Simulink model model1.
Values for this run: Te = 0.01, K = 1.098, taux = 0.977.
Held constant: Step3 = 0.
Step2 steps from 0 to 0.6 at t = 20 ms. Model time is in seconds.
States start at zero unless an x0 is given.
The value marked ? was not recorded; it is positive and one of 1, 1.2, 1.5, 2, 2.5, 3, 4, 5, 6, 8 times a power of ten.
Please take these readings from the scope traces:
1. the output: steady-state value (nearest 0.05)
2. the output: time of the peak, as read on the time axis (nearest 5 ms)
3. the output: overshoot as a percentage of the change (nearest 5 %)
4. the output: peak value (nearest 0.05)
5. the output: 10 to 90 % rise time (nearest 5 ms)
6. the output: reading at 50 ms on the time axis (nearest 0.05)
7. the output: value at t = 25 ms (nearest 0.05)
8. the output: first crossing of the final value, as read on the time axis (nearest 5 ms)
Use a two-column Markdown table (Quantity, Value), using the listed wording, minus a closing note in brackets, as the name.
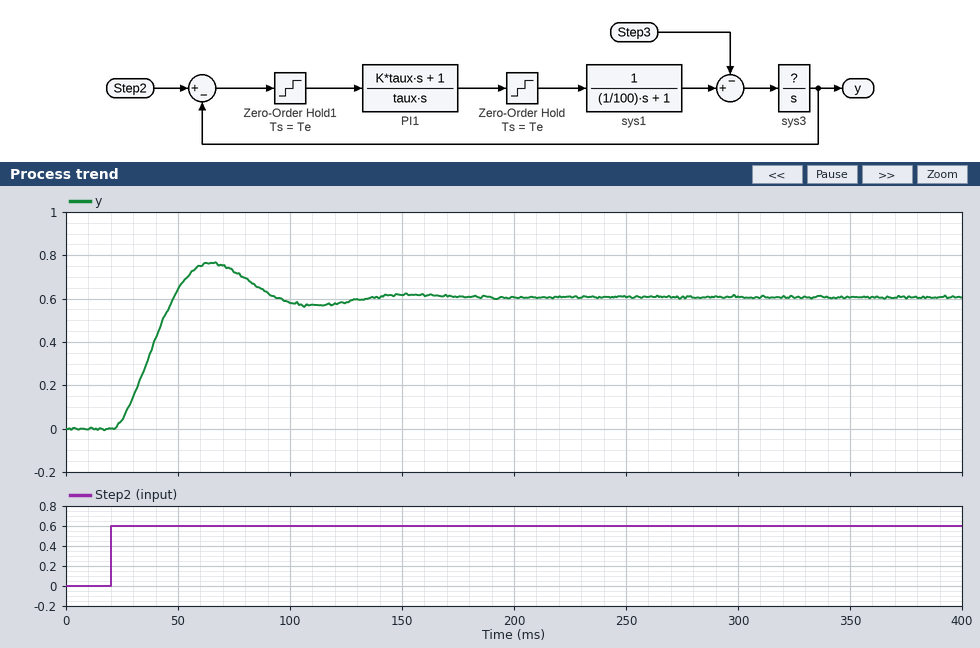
| Quantity | Value |
|---|---|
| the output: steady-state value | 0.60 |
| the output: time of the peak, as read on the time axis | 65 ms |
| the output: overshoot as a percentage of the change | 25 % |
| the output: peak value | 0.75 |
| the output: 10 to 90 % rise time | 20 ms |
| the output: reading at 50 ms on the time axis | 0.65 |
| the output: value at t = 25 ms | 0.05 |
| the output: first crossing of the final value, as read on the time axis | 50 ms |
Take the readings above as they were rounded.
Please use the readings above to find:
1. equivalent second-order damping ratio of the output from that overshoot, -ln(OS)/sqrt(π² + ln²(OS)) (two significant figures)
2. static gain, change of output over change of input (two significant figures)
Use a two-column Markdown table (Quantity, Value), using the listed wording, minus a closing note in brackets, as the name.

| Quantity | Value |
|---|---|
| equivalent second-order damping ratio of the output from that overshoot, -ln(OS)/sqrt(π² + ln²(OS)) | 0.40 |
| static gain, change of output over change of input | 1.0 |
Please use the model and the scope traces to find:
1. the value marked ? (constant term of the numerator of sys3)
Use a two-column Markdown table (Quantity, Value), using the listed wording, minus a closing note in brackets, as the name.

| Quantity | Value |
|---|---|
| the value marked ? | 60 |
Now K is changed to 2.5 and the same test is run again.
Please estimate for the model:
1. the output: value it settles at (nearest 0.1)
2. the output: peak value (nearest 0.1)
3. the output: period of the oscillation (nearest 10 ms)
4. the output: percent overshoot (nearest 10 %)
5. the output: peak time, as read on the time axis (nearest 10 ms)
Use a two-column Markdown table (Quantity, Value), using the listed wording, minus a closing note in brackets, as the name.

| Quantity | Value |
|---|---|
| the output: value it settles at | 0.6 |
| the output: peak value | 1.0 |
| the output: period of the oscillation | 60 ms |
| the output: percent overshoot | 70 % |
| the output: peak time, as read on the time axis | 50 ms |
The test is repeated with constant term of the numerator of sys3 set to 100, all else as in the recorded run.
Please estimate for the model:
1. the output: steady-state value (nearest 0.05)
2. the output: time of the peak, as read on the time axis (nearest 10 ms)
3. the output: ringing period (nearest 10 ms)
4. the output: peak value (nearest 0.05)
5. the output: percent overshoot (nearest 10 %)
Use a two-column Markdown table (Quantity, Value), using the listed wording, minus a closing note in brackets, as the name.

| Quantity | Value |
|---|---|
| the output: steady-state value | 0.60 |
| the output: time of the peak, as read on the time axis | 50 ms |
| the output: ringing period | 70 ms |
| the output: peak value | 0.90 |
| the output: percent overshoot | 50 % |
